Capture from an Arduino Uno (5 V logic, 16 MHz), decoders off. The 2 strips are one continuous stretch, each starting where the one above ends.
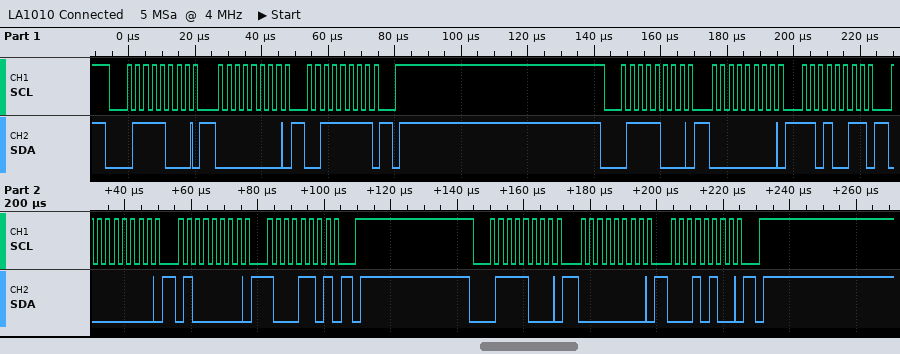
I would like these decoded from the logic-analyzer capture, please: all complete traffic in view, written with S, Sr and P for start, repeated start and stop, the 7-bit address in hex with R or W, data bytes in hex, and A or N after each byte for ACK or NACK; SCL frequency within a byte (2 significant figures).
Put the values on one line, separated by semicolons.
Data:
S 3CW A 00 A 3F A P S 3CW A 00 A D3 A 00 A 40 A 8D A P S 3CW A 00 A 14 A P; 400 kHz
